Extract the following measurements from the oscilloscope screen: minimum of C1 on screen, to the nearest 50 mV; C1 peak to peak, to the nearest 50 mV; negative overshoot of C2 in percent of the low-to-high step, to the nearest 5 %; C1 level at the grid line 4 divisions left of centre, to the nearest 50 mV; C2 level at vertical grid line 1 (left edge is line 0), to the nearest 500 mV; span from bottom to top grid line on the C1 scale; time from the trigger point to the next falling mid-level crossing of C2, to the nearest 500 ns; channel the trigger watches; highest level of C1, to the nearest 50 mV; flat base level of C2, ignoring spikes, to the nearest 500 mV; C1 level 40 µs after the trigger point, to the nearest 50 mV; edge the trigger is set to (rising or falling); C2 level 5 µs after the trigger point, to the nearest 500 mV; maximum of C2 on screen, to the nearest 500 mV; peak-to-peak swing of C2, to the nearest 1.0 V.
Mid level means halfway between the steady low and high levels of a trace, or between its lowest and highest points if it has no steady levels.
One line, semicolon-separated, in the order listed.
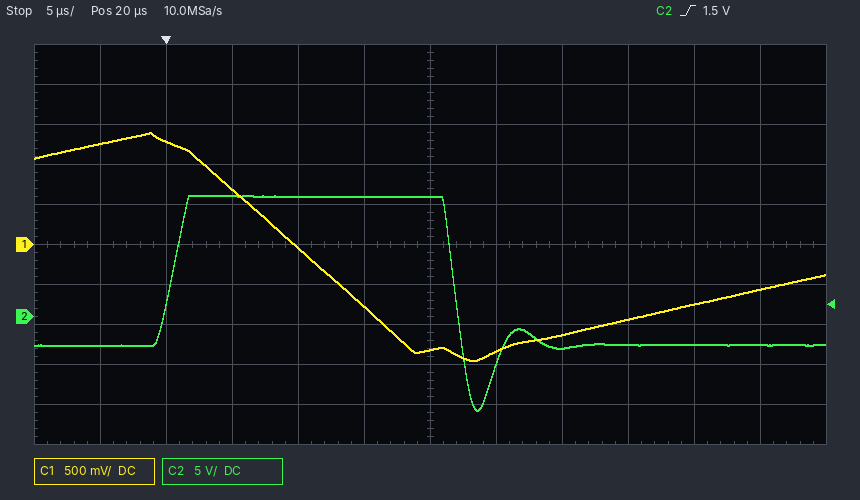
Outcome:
-1.45 V; 2.85 V; 45 %; 1.30 V; -3.5 V; 5 V; 21.5 µs; C2; 1.40 V; -3.5 V; -750 mV; rising; 15.0 V; 15.0 V; 27.0 V
